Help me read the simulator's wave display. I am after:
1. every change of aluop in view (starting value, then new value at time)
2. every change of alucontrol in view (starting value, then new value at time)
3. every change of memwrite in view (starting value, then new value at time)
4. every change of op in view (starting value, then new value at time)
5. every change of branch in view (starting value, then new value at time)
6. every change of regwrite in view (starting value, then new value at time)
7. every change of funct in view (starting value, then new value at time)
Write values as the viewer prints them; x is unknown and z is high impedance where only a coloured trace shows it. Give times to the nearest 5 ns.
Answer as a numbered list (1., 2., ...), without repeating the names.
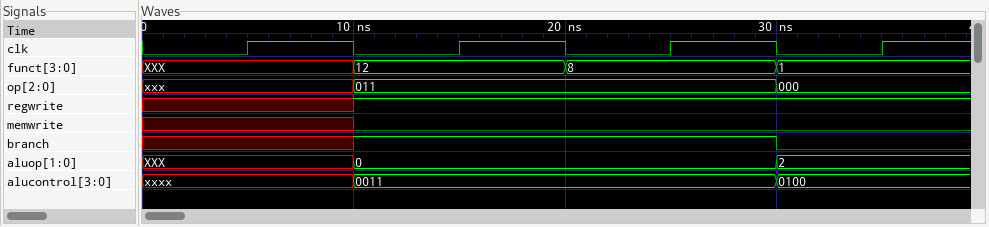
1. XXX, 0 at 10 ns, 2 at 30 ns
2. xxxx, 0011 at 10 ns, 0100 at 30 ns
3. x, 0 at 10 ns
4. xxx, 011 at 10 ns, 000 at 30 ns
5. x, 1 at 10 ns, 0 at 30 ns
6. x, 1 at 10 ns
7. XXX, 12 at 10 ns, 8 at 20 ns, 1 at 30 ns
